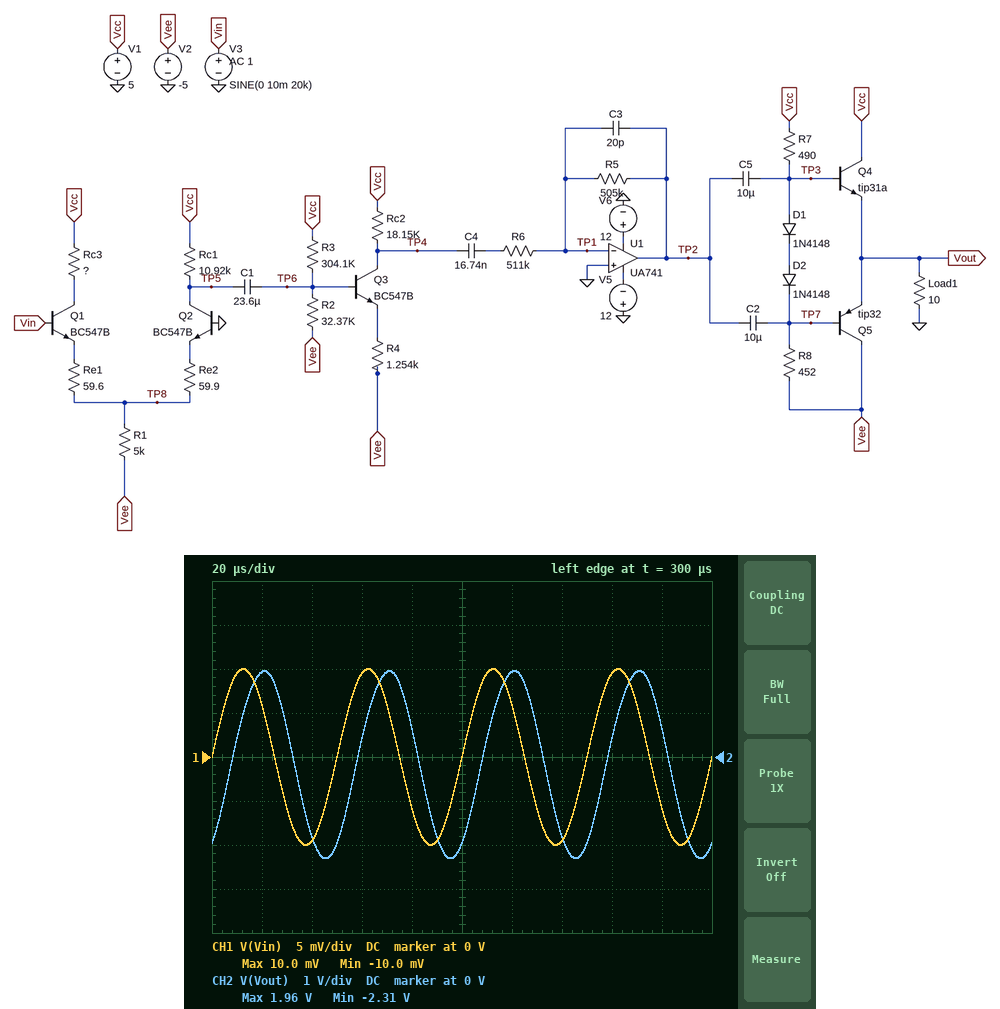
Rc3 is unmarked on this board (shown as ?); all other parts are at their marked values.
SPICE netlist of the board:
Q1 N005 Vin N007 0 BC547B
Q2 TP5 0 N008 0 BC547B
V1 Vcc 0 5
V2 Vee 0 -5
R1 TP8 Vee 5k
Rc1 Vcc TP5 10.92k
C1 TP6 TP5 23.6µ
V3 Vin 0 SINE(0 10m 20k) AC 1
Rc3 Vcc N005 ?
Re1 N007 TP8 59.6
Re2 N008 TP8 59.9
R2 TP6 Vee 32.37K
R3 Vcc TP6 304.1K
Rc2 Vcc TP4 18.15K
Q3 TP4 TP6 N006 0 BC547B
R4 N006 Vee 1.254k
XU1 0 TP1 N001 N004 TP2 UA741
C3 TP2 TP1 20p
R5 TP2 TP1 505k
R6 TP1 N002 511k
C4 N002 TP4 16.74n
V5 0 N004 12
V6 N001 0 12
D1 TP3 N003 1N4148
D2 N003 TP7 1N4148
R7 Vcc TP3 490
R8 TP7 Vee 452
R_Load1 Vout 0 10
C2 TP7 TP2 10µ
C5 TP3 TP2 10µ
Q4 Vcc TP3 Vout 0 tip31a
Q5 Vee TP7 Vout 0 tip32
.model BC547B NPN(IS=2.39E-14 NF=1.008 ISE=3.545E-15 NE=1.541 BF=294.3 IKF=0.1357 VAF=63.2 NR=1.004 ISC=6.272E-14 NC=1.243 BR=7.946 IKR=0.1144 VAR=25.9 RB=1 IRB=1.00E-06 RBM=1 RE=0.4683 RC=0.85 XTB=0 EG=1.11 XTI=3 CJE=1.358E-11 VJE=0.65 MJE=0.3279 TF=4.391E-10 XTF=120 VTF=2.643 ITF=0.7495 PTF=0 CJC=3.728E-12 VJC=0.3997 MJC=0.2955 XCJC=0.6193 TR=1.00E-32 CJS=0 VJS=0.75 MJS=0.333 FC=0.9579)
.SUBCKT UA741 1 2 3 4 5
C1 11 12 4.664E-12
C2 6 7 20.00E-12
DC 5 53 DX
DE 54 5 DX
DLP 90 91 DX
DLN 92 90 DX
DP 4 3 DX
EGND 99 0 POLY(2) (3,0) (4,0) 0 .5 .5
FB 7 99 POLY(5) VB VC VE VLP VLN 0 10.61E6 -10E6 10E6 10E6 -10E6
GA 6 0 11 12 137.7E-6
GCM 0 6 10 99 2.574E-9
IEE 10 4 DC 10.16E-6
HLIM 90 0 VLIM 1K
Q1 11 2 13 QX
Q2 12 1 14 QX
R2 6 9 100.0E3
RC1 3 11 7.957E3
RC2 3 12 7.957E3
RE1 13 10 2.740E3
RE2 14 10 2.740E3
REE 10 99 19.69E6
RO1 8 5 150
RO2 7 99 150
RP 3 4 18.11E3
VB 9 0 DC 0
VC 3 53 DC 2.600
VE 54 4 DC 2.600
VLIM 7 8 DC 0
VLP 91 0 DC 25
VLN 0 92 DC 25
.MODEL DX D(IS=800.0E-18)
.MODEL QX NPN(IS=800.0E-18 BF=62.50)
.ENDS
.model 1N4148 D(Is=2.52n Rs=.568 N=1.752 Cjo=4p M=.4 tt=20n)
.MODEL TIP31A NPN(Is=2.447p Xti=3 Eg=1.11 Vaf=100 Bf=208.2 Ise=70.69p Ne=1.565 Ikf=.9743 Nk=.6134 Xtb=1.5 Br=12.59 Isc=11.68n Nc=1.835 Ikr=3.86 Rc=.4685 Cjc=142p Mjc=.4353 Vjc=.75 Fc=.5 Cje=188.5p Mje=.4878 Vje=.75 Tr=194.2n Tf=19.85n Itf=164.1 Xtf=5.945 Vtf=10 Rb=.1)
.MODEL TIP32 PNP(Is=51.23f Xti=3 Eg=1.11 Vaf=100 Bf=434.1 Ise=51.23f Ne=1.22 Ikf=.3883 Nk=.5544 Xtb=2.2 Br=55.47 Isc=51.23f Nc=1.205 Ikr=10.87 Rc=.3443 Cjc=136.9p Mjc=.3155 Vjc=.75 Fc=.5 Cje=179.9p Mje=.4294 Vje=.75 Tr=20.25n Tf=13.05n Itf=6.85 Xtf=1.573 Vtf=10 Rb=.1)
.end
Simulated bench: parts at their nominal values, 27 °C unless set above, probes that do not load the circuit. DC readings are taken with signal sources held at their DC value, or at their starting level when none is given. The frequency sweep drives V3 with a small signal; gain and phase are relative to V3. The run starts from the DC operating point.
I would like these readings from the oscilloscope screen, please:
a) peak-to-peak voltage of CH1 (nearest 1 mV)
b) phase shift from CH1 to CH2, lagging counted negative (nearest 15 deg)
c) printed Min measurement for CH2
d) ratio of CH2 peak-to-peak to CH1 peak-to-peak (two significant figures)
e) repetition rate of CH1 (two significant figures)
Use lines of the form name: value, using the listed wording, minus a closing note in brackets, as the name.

peak-to-peak voltage of CH1: 20 mV
phase shift from CH1 to CH2, lagging counted negative: -60 deg
printed Min measurement for CH2: -2.31 V
ratio of CH2 peak-to-peak to CH1 peak-to-peak: 210
repetition rate of CH1: 20 kHz
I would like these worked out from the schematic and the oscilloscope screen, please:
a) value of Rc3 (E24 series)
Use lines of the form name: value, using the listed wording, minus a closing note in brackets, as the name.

value of Rc3: 12 kΩ
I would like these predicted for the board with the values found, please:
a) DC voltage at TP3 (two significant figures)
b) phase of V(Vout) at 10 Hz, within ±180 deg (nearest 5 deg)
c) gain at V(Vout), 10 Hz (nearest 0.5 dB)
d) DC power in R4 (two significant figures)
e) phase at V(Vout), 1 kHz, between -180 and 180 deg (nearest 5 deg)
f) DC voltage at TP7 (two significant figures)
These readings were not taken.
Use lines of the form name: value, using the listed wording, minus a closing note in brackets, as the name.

DC voltage at TP3: 540 mV
phase of V(Vout) at 10 Hz, within ±180 deg: 140 deg
gain at V(Vout), 10 Hz: 33.0 dB
DC power in R4: 89 µW
phase at V(Vout), 1 kHz, between -180 and 180 deg: 0 deg
DC voltage at TP7: -830 mV
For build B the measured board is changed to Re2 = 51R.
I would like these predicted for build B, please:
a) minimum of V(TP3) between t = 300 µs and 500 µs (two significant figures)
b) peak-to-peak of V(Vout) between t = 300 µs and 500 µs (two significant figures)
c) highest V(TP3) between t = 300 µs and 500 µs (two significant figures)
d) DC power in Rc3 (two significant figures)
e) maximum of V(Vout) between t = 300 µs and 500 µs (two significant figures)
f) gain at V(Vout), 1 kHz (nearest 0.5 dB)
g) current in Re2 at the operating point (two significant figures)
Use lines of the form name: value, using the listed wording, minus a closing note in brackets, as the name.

minimum of V(TP3) between t = 300 µs and 500 µs: -1.8 V
peak-to-peak of V(Vout) between t = 300 µs and 500 µs: 4.7 V
highest V(TP3) between t = 300 µs and 500 µs: 3.0 V
DC power in Rc3: 2.1 mW
maximum of V(Vout) between t = 300 µs and 500 µs: 2.3 V
gain at V(Vout), 1 kHz: 52.0 dB
current in Re2 at the operating point: 450 µA
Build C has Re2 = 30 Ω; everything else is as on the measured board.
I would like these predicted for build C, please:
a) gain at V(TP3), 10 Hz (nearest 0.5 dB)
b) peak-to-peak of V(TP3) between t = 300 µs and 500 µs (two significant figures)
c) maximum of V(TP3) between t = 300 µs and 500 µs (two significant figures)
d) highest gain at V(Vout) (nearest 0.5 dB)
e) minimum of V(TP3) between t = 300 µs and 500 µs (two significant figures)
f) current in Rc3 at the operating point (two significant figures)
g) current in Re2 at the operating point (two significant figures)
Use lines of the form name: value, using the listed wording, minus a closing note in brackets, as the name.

gain at V(TP3), 10 Hz: 34.0 dB
peak-to-peak of V(TP3) between t = 300 µs and 500 µs: 4.2 V
maximum of V(TP3) between t = 300 µs and 500 µs: 3.3 V
highest gain at V(Vout): 52.5 dB
minimum of V(TP3) between t = 300 µs and 500 µs: -880 mV
current in Rc3 at the operating point: 380 µA
current in Re2 at the operating point: 500 µA
